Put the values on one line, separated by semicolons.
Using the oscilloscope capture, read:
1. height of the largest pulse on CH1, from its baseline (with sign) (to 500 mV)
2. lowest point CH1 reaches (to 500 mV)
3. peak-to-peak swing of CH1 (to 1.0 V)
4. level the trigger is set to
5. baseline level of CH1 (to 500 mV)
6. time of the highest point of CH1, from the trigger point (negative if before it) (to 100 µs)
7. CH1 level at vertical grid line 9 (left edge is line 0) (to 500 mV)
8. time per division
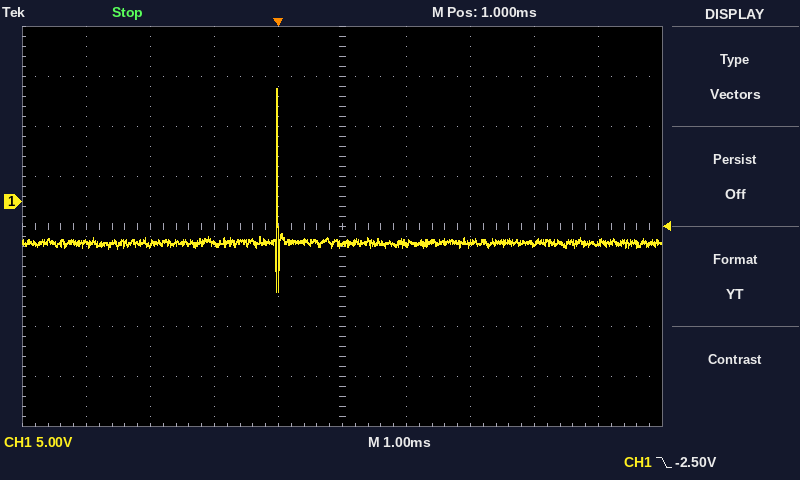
+15.5 V; -9.0 V; 20.0 V; -2.50 V; -4.0 V; 0.0 ms; -4.0 V; 1 ms
